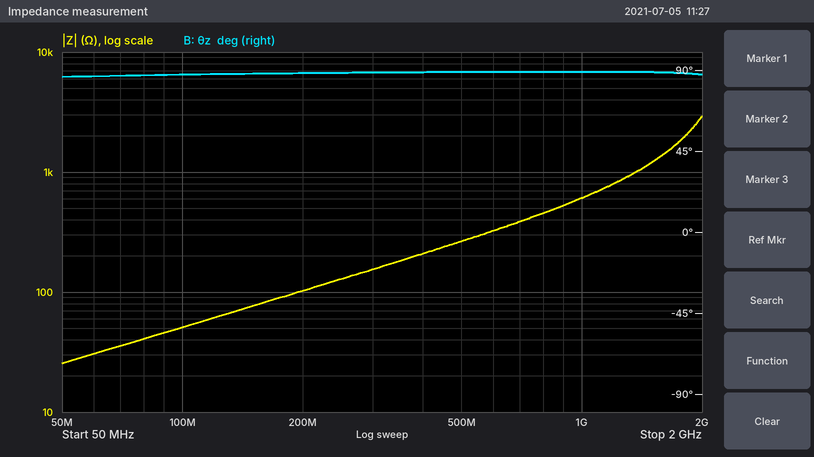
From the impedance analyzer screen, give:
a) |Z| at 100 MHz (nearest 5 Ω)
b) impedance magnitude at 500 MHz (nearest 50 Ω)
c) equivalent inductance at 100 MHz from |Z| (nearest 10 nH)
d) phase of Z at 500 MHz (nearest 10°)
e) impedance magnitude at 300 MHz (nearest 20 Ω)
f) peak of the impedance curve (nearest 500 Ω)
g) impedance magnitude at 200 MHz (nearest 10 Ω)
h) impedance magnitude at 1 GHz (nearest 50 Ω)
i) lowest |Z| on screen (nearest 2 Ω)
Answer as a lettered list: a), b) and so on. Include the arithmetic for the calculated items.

a) 50 Ω
b) 250 Ω
c) L = 50 Ω/(2π × 100 MHz) ≈ 80 nH
d) 90°
e) 160 Ω
f) 3.0 kΩ
g) 100 Ω
h) 600 Ω
i) 26 Ω
